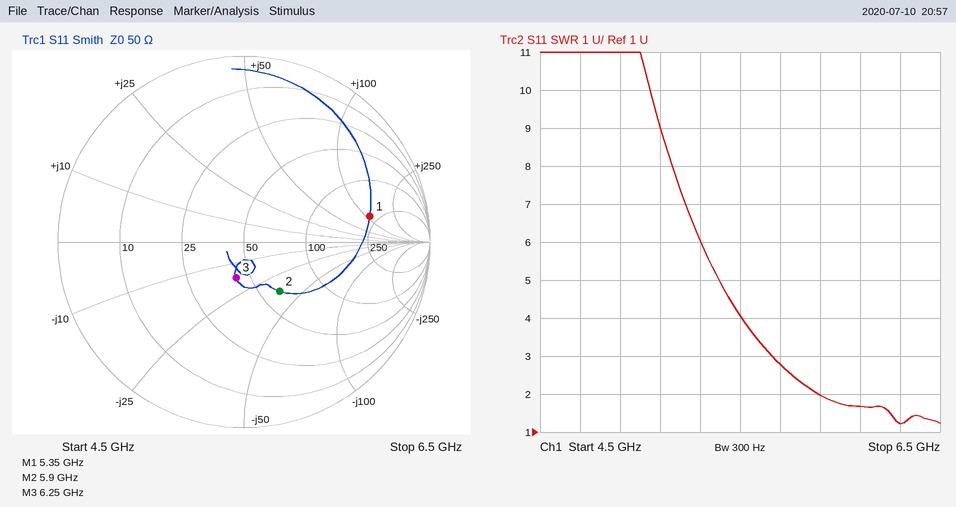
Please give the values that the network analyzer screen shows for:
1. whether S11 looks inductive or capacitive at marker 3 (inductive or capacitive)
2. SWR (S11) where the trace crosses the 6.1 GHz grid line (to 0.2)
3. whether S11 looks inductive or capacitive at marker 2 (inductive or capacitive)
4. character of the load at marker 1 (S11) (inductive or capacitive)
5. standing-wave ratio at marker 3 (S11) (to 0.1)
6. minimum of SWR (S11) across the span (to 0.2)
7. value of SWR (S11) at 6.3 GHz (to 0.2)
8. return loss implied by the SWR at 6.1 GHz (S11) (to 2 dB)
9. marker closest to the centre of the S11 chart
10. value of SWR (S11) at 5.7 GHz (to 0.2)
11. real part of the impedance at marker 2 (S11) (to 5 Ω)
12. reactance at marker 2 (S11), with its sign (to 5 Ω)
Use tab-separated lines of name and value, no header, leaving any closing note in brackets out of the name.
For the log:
whether S11 looks inductive or capacitive at marker 3	capacitive
SWR (S11) where the trace crosses the 6.1 GHz grid line	1.6
whether S11 looks inductive or capacitive at marker 2	capacitive
character of the load at marker 1 (S11)	inductive
standing-wave ratio at marker 3 (S11)	1.5
minimum of SWR (S11) across the span	1.2
value of SWR (S11) at 6.3 GHz	1.2
return loss implied by the SWR at 6.1 GHz (S11)	12 dB
marker closest to the centre of the S11 chart	marker 3
value of SWR (S11) at 5.7 GHz	2.8
real part of the impedance at marker 2 (S11)	60 Ω
reactance at marker 2 (S11), with its sign	-35 Ω
